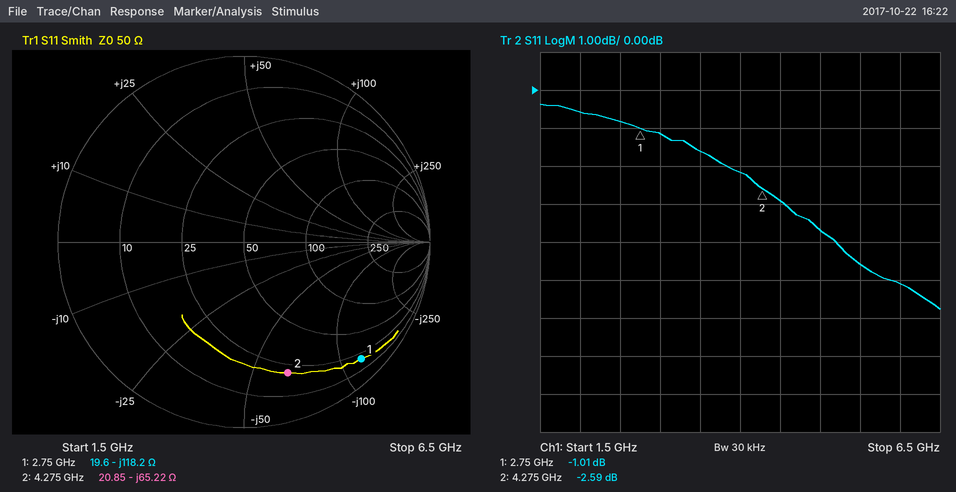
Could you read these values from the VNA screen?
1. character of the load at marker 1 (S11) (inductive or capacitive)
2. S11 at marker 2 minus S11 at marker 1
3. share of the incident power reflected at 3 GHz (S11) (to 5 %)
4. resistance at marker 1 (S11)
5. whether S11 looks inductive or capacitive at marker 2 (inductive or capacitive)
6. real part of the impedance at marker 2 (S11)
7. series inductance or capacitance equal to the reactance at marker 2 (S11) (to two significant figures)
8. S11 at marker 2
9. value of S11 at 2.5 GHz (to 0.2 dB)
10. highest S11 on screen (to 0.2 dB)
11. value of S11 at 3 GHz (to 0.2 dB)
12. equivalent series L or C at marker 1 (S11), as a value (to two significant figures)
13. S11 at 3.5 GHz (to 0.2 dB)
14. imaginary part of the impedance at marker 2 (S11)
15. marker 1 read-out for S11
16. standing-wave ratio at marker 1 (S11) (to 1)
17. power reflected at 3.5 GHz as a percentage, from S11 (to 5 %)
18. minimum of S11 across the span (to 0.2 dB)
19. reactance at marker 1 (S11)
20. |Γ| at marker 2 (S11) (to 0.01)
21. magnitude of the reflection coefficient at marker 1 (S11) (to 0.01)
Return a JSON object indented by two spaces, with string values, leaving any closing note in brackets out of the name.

{
  "character of the load at marker 1 (S11)": "capacitive",
  "S11 at marker 2 minus S11 at marker 1": "-1.58 dB",
  "share of the incident power reflected at 3 GHz (S11)": "75 %",
  "resistance at marker 1": "19.6 Ω",
  "whether S11 looks inductive or capacitive at marker 2": "capacitive",
  "real part of the impedance at marker 2": "20.85 Ω",
  "series inductance or capacitance equal to the reactance at marker 2 (S11)": "570 fF",
  "S11 at marker 2": "-2.59 dB",
  "value of S11 at 2.5 GHz": "-0.8 dB",
  "highest S11 on screen": "-0.4 dB",
  "value of S11 at 3 GHz": "-1.2 dB",
  "equivalent series L or C at marker 1 (S11), as a value": "490 fF",
  "S11 at 3.5 GHz": "-1.6 dB",
  "imaginary part of the impedance at marker 2": "-65.22 Ω",
  "marker 1 read-out for S11": "-1.01 dB",
  "standing-wave ratio at marker 1 (S11)": "17",
  "power reflected at 3.5 GHz as a percentage, from S11": "70 %",
  "minimum of S11 across the span": "-5.8 dB",
  "reactance at marker 1": "-118.2 Ω",
  "|Γ| at marker 2 (S11)": "0.74",
  "magnitude of the reflection coefficient at marker 1 (S11)": "0.89"
}
